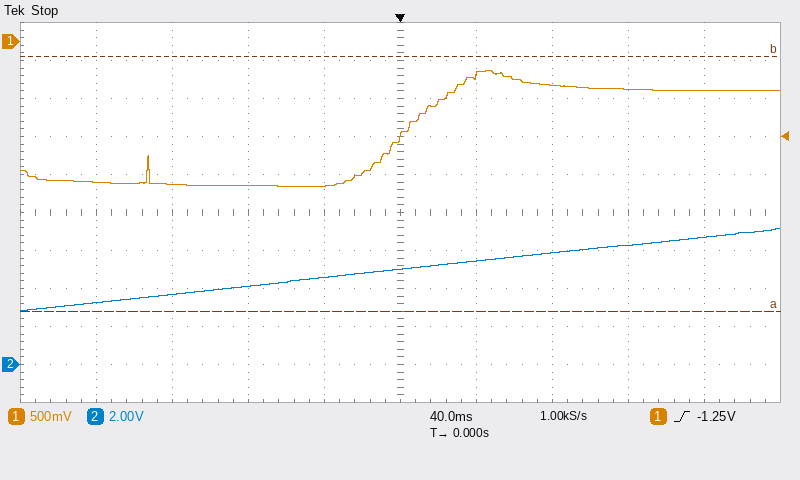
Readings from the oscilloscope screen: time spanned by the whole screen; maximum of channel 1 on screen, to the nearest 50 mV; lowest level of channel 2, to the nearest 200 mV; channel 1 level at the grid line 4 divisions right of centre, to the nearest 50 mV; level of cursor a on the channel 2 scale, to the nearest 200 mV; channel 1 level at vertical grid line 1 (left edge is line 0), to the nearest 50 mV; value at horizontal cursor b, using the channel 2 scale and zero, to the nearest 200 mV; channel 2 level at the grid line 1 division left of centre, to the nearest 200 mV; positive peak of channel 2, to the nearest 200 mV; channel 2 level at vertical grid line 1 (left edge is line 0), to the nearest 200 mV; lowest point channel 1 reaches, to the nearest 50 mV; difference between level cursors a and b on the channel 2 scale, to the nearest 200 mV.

400 ms
-400 mV
2.8 V
-650 mV
2.8 V
-1.85 V
16.2 V
4.6 V
7.2 V
3.2 V
-1.90 V
13.4 V
